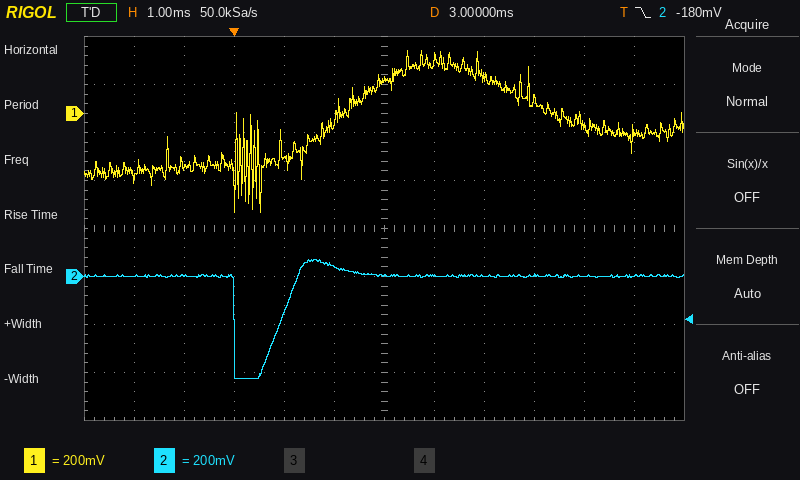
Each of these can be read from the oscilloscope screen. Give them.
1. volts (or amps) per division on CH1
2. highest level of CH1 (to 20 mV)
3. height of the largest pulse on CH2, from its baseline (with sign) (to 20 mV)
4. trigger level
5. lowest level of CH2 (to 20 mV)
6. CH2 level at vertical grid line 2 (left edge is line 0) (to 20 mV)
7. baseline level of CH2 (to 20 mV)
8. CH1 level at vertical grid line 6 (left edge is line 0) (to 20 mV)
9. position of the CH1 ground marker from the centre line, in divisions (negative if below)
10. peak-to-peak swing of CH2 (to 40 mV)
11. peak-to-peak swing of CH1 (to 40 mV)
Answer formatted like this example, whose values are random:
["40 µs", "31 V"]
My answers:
["200 mV", "260 mV", "-420 mV", "-180 mV", "-420 mV", "0 mV", "0 mV", "140 mV", "+2.4 div", "480 mV", "680 mV"]
